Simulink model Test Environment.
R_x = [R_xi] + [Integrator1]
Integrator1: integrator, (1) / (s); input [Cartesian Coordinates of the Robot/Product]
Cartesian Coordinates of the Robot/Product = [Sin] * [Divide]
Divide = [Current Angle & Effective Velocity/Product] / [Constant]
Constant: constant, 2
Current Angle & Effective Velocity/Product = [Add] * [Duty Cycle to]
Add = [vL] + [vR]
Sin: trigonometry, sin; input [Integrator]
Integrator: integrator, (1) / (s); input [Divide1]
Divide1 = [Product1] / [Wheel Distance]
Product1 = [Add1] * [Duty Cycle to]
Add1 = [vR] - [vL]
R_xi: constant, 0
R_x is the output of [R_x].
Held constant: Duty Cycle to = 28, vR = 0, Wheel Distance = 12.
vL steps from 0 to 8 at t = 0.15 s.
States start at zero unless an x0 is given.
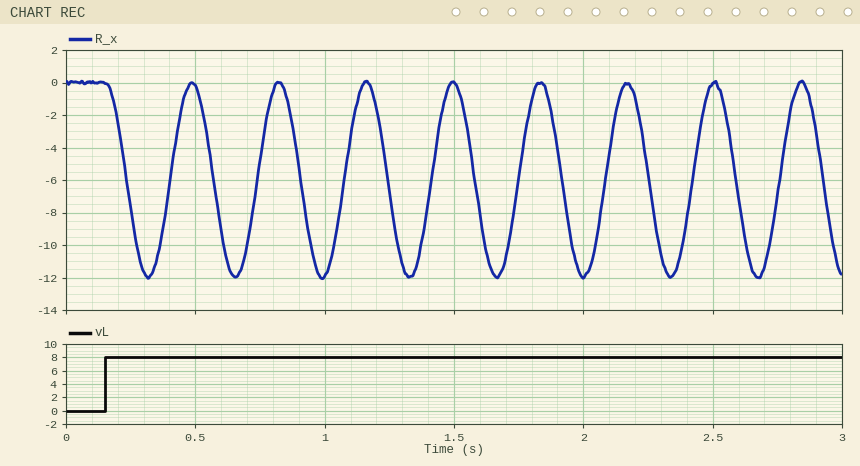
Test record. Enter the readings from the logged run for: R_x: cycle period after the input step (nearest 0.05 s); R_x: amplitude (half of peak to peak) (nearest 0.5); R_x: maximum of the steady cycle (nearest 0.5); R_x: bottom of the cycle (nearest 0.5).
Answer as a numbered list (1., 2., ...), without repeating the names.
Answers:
1. 0.35 s
2. 6.0
3. 0.0
4. -12.0
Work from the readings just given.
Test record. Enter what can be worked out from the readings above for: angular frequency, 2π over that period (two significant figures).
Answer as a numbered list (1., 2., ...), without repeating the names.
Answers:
1. 18 rad/s
